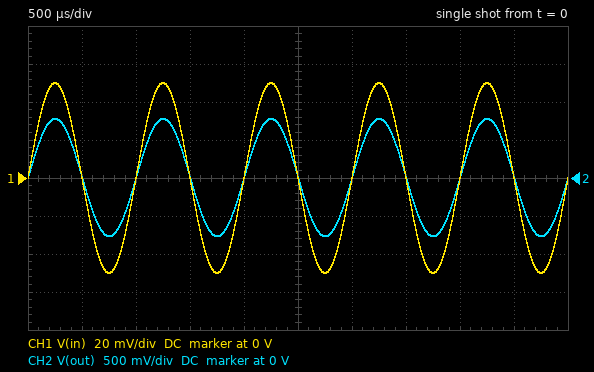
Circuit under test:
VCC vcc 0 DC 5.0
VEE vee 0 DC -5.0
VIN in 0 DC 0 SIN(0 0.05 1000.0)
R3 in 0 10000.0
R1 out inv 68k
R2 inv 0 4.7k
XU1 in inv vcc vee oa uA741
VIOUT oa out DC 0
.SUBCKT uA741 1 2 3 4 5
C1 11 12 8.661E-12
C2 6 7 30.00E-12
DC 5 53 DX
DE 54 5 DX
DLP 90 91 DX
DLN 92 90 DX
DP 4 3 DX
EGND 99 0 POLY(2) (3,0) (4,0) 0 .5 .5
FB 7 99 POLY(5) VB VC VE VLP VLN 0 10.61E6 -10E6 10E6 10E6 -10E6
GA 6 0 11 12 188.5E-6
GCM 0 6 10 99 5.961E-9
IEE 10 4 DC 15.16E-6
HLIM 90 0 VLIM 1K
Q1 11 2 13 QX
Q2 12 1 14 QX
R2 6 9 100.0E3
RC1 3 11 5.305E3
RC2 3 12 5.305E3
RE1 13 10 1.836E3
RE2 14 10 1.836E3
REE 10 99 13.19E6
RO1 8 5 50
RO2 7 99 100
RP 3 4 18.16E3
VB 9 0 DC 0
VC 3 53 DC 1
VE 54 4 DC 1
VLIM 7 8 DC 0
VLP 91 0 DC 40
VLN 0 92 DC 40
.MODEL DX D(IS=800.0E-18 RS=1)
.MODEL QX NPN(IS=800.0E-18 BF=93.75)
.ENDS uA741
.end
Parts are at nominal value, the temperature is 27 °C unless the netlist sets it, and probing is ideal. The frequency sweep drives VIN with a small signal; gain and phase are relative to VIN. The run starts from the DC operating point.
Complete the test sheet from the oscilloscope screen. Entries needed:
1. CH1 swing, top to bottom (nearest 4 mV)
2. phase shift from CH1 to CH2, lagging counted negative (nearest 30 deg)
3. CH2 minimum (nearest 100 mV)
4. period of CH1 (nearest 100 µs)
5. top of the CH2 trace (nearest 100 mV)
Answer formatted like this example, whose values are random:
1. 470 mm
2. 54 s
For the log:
1. 100 mV
2. 0 deg
3. -800 mV
4. 1.0 ms
5. 800 mV
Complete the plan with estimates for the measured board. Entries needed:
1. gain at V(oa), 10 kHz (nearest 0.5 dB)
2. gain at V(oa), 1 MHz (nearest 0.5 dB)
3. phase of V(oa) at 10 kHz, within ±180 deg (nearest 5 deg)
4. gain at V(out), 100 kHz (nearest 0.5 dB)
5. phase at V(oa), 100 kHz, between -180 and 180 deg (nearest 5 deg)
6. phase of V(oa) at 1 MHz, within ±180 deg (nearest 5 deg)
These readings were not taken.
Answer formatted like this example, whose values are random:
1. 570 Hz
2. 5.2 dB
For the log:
1. 23.5 dB
2. -1.0 dB
3. -10 deg
4. 18.5 dB
5. -60 deg
6. -115 deg
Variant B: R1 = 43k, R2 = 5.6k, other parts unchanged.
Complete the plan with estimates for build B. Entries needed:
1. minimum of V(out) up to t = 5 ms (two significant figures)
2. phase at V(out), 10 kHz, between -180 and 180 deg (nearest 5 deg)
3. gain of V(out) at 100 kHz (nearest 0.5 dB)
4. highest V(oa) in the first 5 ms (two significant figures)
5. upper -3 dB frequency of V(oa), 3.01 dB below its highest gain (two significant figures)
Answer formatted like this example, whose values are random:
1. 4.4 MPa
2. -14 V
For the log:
1. -430 mV
2. -5 deg
3. 16.5 dB
4. 440 mV
5. 120 kHz
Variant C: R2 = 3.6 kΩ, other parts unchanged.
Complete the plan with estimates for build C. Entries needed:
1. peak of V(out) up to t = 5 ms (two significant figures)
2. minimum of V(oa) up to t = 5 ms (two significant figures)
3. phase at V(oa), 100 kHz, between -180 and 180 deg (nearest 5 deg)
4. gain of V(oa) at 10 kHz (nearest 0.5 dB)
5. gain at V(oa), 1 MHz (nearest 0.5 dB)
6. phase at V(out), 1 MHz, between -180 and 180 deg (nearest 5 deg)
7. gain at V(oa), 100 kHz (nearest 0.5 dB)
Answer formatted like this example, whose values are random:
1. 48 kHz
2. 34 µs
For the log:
1. 1.0 V
2. -990 mV
3. -65 deg
4. 26.0 dB
5. -1.0 dB
6. -120 deg
7. 19.0 dB
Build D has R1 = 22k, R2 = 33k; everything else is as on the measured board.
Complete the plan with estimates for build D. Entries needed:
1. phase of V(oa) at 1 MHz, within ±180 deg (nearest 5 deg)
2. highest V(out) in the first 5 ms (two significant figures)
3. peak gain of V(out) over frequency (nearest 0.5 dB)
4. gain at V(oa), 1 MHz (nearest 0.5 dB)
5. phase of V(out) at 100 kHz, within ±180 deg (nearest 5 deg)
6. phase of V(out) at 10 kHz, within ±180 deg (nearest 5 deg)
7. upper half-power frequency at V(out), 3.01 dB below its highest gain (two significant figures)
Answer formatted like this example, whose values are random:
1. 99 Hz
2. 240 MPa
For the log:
1. -90 deg
2. 85 mV
3. 4.5 dB
4. 0 dB
5. -10 deg
6. 0 deg
7. 810 kHz
